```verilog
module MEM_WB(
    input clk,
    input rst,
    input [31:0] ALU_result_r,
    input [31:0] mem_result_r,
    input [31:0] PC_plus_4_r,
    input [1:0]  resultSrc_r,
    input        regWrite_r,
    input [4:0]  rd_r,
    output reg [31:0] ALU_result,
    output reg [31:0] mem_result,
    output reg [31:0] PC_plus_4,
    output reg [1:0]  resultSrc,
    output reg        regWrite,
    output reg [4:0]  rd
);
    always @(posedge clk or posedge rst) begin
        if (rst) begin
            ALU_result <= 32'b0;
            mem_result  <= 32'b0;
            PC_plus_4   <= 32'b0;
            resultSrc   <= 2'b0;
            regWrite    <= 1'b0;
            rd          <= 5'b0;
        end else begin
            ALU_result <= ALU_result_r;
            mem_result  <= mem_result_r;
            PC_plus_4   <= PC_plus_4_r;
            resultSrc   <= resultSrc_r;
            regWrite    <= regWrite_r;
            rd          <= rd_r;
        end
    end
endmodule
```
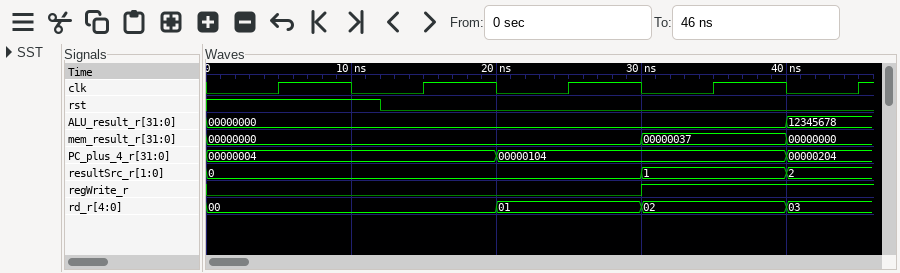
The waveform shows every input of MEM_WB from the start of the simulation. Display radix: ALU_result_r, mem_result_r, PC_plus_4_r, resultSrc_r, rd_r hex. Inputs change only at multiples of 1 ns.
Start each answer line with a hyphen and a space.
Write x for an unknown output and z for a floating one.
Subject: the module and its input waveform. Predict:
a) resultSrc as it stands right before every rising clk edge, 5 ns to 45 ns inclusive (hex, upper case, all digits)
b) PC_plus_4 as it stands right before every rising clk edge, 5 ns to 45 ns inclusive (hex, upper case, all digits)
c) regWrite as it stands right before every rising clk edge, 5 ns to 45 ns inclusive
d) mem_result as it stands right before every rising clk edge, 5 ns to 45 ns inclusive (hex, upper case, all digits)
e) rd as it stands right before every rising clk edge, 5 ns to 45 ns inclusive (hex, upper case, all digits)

- 0, 0, 0, 0, 1
- 00000000, 00000000, 00000004, 00000104, 00000104
- 0 0 0 0 1
- 00000000, 00000000, 00000000, 00000000, 00000037
- 00, 00, 00, 01, 02
